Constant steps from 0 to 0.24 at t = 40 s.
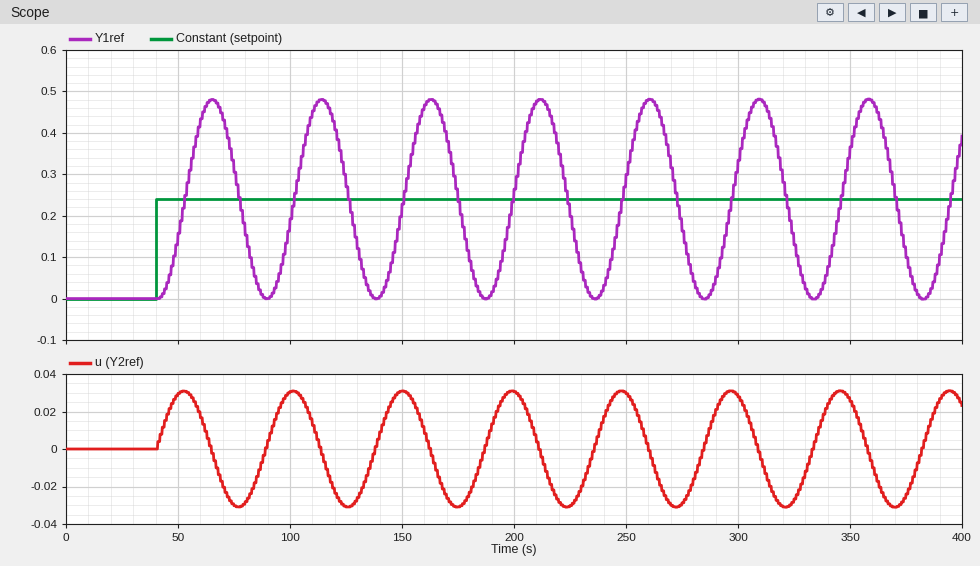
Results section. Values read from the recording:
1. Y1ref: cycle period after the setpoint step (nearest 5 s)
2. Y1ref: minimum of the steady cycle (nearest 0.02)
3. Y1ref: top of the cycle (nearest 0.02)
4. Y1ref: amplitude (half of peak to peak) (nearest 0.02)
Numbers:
50 s
0.00
0.48
0.24
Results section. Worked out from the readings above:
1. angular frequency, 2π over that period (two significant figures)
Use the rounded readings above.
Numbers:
0.13 rad/s
